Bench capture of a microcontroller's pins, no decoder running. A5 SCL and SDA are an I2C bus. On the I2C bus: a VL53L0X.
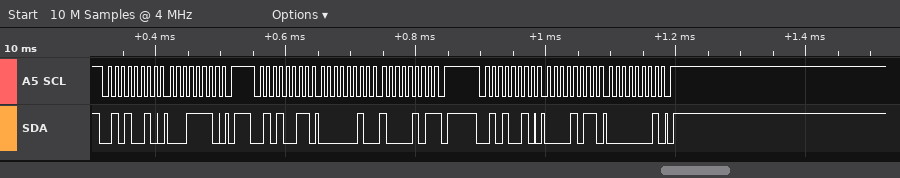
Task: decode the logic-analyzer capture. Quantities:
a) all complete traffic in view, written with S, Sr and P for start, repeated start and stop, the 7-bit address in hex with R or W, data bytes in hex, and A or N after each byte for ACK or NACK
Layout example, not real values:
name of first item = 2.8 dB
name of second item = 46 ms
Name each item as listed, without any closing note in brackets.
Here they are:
all complete traffic in view, written with S, Sr and P for start, repeated start and stop, the 7-bit address in hex with R or W, data bytes in hex, and A or N after each byte for ACK or NACK = S 29W A 1E A P S 29R A 02 A 85 N P S 29W A 0B A 01 A P
